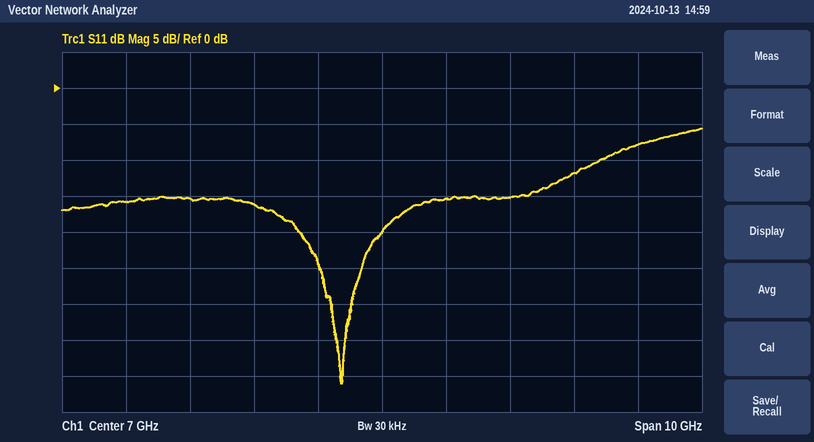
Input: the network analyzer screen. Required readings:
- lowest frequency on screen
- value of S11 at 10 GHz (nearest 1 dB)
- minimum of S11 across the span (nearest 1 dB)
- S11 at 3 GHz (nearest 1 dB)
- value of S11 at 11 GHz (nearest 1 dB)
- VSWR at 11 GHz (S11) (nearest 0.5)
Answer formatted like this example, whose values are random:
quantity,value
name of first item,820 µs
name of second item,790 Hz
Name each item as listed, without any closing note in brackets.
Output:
quantity,value
lowest frequency on screen,2 GHz
value of S11 at 10 GHz,-12 dB
minimum of S11 across the span,-41 dB
S11 at 3 GHz,-16 dB
value of S11 at 11 GHz,-8 dB
VSWR at 11 GHz (S11),2.5
